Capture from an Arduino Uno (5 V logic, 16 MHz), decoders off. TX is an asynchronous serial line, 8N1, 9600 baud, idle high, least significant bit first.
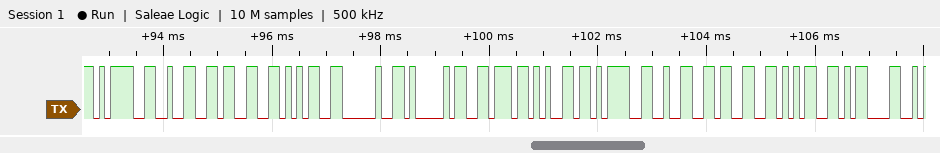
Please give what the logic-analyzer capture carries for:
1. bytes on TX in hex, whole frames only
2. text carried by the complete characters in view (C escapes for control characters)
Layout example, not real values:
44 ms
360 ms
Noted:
3D 32 33 35 20 41 76 65 3D 32 33 35 0D
"=235 Ave=235\r"
